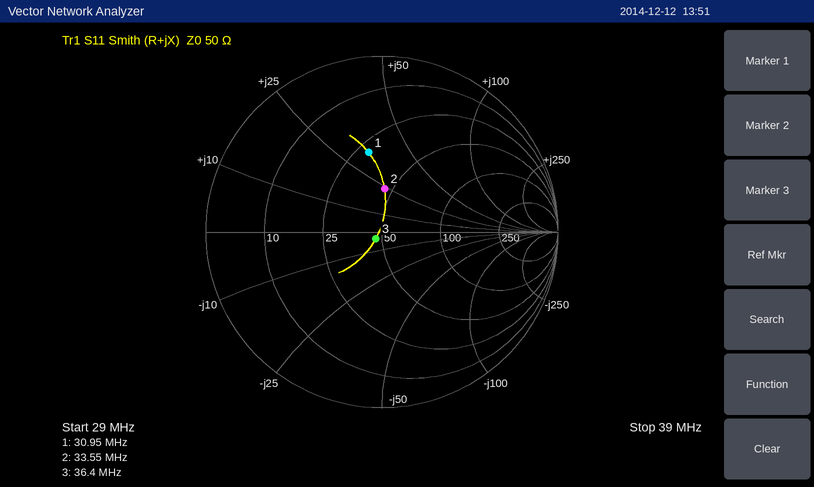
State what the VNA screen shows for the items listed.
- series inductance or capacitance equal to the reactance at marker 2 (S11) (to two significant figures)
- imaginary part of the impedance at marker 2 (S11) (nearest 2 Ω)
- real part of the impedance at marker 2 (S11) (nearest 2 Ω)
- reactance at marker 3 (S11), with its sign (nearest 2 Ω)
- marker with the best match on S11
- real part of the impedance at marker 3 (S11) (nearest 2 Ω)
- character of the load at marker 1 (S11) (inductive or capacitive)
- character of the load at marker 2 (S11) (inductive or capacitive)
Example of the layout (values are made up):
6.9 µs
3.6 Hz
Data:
110 nH
+24 Ω
46 Ω
-4 Ω
marker 3
46 Ω
inductive
inductive
